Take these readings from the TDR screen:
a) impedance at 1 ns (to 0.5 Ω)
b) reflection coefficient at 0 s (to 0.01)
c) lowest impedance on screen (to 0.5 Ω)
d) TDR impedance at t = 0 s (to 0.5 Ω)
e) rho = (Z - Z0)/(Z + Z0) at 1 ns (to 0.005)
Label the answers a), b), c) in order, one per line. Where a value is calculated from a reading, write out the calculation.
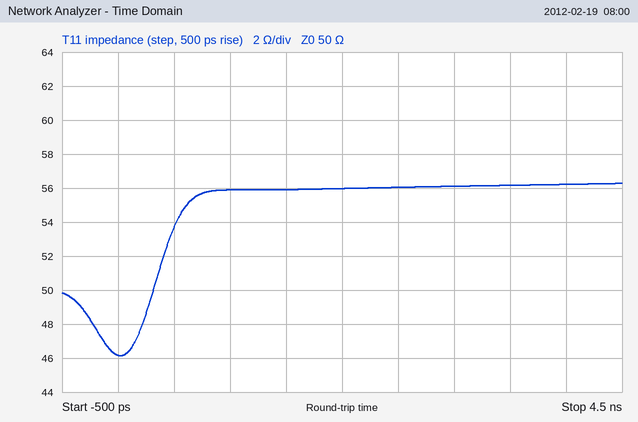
a) 56.0 Ω
b) (46 − 50)/(46 + 50) ≈ -0.04
c) 46.0 Ω
d) 46.0 Ω
e) (56 − 50)/(56 + 50) ≈ +0.0566, so +0.055 to the nearest 0.005
